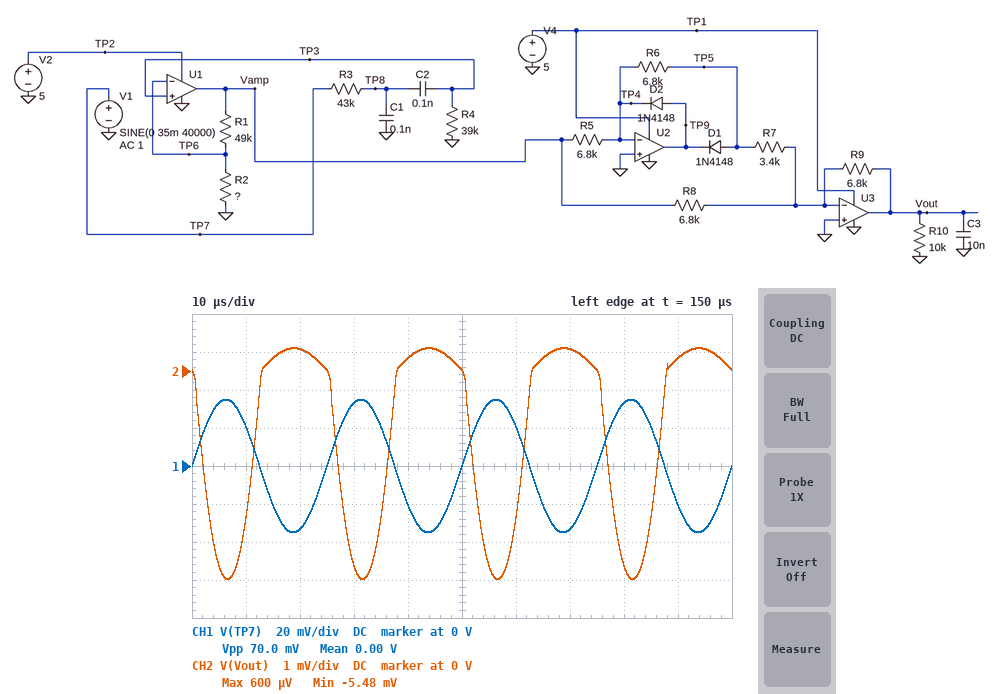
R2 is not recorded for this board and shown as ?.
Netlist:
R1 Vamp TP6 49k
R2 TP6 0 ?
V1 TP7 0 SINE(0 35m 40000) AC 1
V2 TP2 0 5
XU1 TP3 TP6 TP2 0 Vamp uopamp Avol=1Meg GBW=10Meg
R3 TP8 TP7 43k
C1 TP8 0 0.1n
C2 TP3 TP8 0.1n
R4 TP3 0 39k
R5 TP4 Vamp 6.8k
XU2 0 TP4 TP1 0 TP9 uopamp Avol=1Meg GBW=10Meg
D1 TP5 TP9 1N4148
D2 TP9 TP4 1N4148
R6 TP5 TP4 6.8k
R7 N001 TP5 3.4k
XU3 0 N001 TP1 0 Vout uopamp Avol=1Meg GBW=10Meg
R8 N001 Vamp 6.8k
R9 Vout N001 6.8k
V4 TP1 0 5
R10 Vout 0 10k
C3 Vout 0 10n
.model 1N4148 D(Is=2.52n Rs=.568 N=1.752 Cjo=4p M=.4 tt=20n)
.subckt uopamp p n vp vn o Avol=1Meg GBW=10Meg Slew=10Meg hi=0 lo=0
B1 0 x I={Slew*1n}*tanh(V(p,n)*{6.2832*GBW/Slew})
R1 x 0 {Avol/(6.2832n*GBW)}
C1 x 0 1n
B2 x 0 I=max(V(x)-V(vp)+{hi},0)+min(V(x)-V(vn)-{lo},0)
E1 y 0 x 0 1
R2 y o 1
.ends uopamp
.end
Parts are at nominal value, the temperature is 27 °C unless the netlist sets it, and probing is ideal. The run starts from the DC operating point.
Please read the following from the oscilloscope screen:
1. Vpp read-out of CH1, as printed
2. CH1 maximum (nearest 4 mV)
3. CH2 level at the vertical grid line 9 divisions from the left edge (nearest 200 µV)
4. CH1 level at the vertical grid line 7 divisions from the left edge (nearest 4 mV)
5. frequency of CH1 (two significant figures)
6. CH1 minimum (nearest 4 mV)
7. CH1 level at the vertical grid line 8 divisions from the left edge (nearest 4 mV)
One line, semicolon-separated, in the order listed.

70.0 mV; 36 mV; 400 µV; -32 mV; 40 kHz; -36 mV; 32 mV
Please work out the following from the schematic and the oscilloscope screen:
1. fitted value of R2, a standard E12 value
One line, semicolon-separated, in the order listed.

3.3 kΩ
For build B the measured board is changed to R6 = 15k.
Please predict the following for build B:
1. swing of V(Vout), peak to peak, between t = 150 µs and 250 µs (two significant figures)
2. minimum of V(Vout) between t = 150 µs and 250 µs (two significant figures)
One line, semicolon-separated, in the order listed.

5.8 mV; -5.3 mV
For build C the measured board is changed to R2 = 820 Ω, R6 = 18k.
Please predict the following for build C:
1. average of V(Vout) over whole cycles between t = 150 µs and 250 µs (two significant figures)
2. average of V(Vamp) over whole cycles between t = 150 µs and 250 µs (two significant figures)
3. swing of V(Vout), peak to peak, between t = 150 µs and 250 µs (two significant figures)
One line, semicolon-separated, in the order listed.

-3.8 mV; 210 mV; 10 mV
